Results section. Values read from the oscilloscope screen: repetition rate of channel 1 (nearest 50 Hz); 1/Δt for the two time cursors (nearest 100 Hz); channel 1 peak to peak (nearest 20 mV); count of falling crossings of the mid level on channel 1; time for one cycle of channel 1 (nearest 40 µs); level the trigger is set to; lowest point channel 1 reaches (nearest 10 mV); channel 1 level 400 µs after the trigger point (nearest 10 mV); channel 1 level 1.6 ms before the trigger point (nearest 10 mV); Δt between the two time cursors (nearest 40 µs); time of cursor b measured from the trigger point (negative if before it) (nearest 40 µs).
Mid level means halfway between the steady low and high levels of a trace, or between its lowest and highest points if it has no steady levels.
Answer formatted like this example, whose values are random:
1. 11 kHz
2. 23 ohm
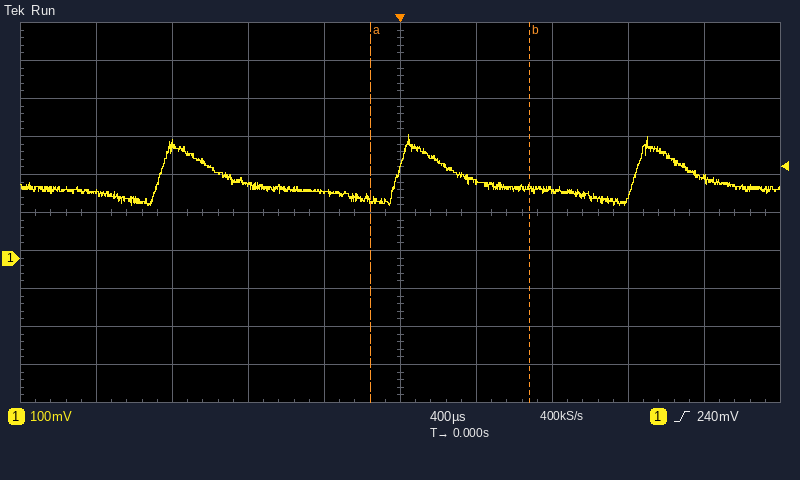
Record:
1. 800 Hz
2. 1.2 kHz
3. 180 mV
4. 3
5. 1.24 ms
6. 240 mV
7. 140 mV
8. 200 mV
9. 170 mV
10. 840 µs
11. +680 µs
